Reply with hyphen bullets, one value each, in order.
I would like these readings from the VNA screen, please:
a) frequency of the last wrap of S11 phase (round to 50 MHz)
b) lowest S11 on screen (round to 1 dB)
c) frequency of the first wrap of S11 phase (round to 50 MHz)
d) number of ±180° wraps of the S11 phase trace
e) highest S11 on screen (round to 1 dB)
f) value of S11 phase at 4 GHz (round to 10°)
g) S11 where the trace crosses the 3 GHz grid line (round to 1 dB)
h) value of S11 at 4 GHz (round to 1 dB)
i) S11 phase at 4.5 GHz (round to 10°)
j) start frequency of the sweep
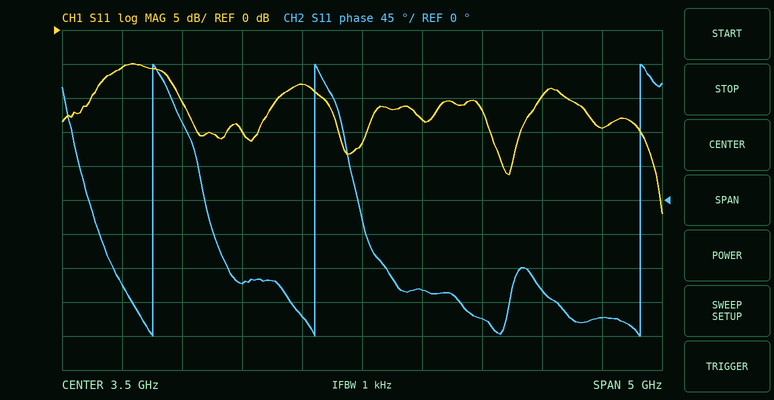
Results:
- 5.80 GHz
- -27 dB
- 1.75 GHz
- 3
- -5 dB
- -120°
- -8 dB
- -13 dB
- -160°
- 1 GHz
